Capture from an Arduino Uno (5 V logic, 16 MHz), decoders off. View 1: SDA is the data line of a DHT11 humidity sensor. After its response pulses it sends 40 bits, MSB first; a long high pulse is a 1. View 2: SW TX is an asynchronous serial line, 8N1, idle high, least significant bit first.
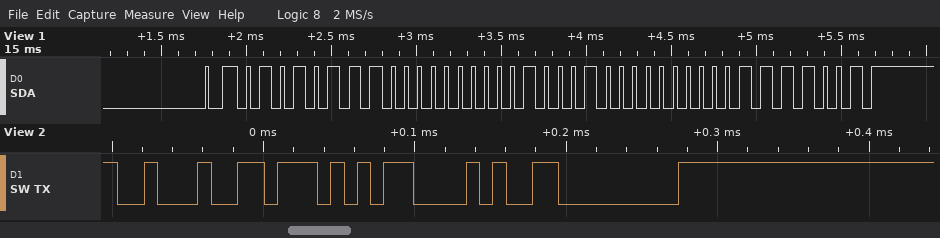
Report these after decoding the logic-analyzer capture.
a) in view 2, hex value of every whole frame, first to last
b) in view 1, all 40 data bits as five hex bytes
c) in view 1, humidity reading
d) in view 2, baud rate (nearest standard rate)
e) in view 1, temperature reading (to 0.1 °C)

22 57 28 00
57 00 22 00 79
87 %
115200 baud
34.0 °C
